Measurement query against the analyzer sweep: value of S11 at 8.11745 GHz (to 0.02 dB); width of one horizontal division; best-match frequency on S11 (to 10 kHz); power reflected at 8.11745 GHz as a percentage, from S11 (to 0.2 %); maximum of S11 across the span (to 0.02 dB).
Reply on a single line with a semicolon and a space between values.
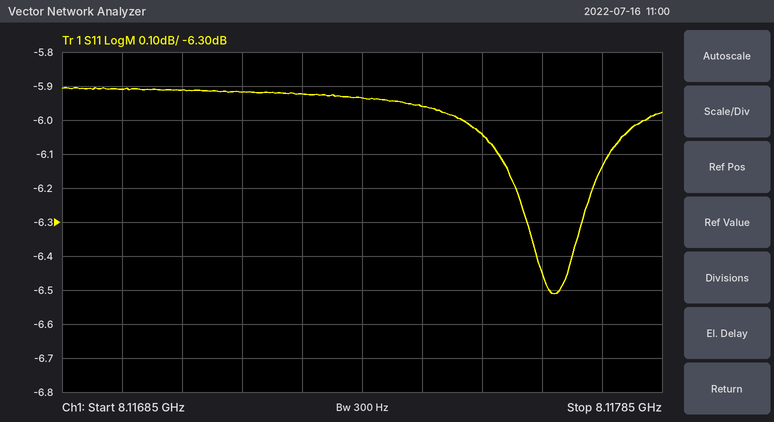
-5.96 dB; 100 kHz; 8.11767 GHz; 25.4 %; -5.90 dB
